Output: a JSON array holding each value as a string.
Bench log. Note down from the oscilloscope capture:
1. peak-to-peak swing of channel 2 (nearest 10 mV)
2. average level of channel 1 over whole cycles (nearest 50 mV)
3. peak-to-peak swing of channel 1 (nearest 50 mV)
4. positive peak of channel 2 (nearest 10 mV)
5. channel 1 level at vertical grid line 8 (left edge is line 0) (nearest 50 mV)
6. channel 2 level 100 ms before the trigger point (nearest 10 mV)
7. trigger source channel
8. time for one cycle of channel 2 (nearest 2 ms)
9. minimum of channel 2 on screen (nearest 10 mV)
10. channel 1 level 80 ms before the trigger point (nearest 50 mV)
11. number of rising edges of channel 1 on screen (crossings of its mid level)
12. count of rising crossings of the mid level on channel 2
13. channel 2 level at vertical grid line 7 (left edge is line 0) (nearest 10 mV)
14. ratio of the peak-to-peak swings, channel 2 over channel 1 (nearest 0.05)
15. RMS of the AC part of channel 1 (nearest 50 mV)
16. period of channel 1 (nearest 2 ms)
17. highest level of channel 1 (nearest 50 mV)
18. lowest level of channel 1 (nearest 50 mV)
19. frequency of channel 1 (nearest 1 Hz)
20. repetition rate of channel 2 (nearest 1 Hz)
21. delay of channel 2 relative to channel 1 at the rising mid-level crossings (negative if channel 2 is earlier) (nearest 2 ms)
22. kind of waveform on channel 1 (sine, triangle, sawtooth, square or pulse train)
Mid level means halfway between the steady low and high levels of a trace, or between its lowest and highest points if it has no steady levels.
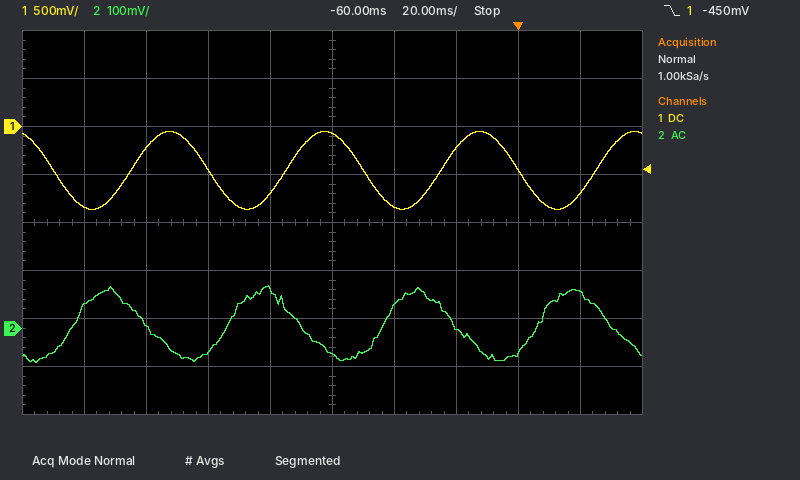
["160 mV", "-450 mV", "800 mV", "90 mV", "-450 mV", "-50 mV", "channel 1", "50 ms", "-70 mV", "-700 mV", "4", "4", "0 mV", "0.20", "300 mV", "50 ms", "-50 mV", "-850 mV", "20 Hz", "20 Hz", "-18 ms", "sine"]
